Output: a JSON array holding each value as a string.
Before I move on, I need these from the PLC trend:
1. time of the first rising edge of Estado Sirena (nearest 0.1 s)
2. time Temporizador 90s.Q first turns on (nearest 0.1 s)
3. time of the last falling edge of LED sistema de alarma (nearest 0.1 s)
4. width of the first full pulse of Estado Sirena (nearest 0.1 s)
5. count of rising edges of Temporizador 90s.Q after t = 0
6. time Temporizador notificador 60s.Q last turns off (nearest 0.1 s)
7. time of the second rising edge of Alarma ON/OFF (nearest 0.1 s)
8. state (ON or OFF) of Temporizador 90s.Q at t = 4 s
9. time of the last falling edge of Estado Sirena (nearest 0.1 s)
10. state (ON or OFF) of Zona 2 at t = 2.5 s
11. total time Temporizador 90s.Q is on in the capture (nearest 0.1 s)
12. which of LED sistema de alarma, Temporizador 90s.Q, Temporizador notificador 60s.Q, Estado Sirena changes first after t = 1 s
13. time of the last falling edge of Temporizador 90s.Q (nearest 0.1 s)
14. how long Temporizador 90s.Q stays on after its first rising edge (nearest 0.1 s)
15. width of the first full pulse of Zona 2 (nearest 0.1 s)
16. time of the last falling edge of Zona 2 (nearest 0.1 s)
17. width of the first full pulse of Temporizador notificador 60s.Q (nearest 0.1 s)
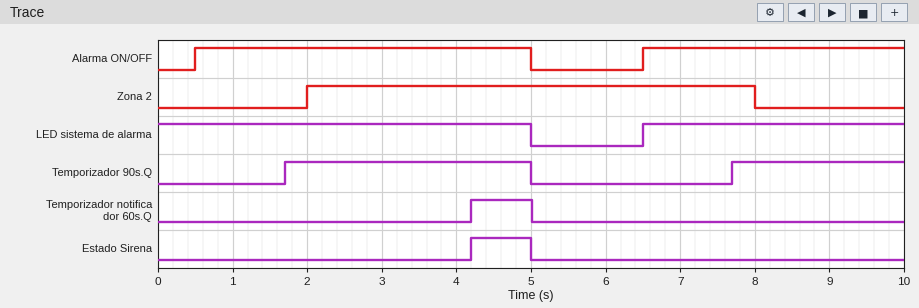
["4.2 s", "1.7 s", "5.0 s", "0.8 s", "2", "5.0 s", "6.5 s", "ON", "5.0 s", "ON", "5.6 s", "Temporizador 90s.Q", "5.0 s", "3.3 s", "6.0 s", "8.0 s", "0.8 s"]
